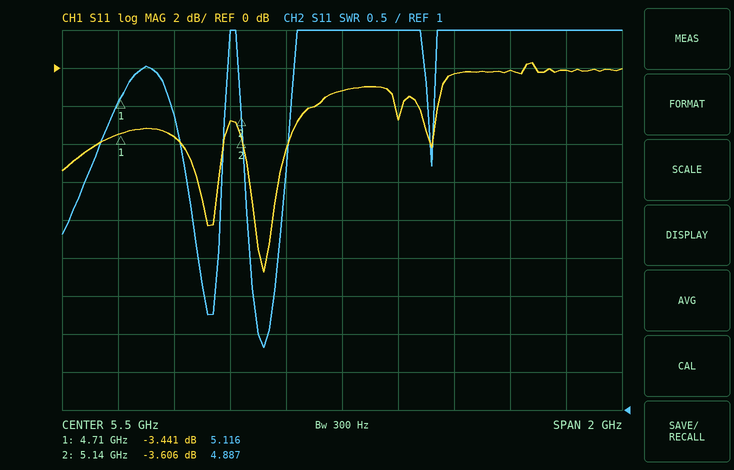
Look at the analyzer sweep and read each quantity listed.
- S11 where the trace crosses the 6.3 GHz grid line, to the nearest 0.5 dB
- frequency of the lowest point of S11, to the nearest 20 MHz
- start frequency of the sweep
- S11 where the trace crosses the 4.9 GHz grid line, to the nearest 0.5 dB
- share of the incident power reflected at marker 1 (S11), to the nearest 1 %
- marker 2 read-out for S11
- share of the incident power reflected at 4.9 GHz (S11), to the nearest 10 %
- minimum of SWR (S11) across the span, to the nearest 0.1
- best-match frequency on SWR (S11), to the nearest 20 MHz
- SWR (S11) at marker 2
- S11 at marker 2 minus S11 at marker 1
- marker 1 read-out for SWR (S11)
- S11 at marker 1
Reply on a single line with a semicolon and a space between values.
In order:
0.0 dB; 5.22 GHz; 4.5 GHz; -3.5 dB; 45 %; -3.606 dB; 40 %; 1.8; 5.22 GHz; 4.887; -0.165 dB; 5.116; -3.441 dB
